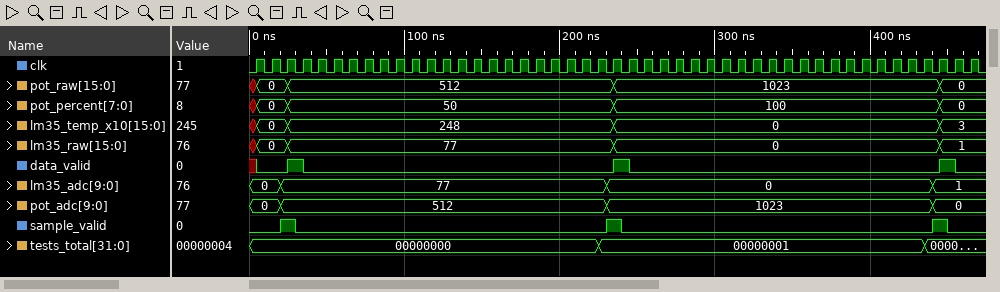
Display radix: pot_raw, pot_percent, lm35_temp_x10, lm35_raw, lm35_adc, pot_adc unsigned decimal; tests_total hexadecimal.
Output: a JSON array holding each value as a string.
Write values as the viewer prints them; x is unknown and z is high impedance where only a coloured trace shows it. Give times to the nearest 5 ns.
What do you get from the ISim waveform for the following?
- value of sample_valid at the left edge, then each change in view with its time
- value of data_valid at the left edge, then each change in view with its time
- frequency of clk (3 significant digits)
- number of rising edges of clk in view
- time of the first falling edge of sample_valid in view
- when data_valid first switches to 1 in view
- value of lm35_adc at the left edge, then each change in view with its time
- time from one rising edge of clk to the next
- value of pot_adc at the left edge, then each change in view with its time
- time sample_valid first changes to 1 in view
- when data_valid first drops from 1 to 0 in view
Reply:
["0, 1 at 20 ns, 0 at 30 ns, 1 at 230 ns, 0 at 240 ns, 1 at 440 ns, 0 at 450 ns", "x, 0 at 5 ns, 1 at 25 ns, 0 at 35 ns, 1 at 235 ns, 0 at 245 ns, 1 at 445 ns, 0 at 455 ns", "100 MHz", "47", "30 ns", "25 ns", "0, 77 at 20 ns, 0 at 230 ns, 1 at 440 ns", "10 ns", "0, 512 at 20 ns, 1023 at 230 ns, 0 at 440 ns", "20 ns", "35 ns"]
